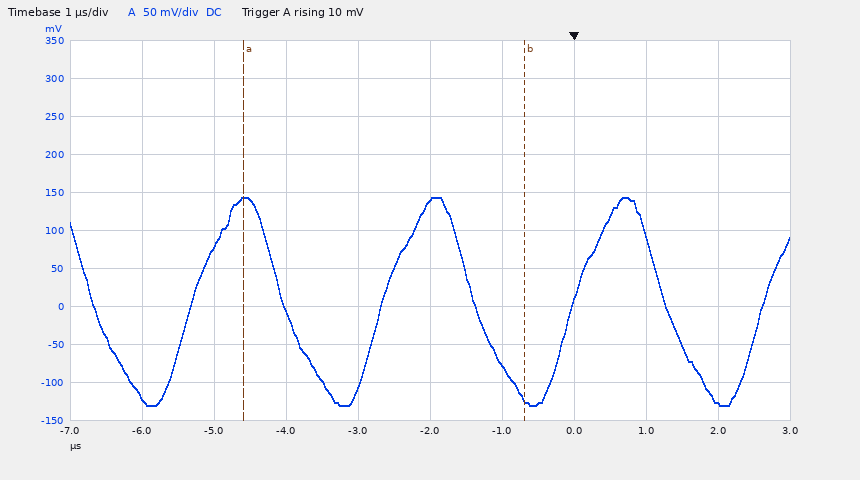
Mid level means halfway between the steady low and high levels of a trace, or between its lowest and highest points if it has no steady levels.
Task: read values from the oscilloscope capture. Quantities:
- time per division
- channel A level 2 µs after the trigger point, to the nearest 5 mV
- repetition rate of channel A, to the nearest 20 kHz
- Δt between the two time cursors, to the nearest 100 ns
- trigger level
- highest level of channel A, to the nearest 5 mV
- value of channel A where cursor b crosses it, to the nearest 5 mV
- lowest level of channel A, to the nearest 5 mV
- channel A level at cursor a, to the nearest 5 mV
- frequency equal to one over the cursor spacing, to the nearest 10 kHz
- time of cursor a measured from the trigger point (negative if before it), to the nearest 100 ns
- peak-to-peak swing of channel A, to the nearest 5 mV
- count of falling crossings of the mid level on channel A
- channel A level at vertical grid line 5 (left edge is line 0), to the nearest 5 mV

1 µs
-130 mV
380 kHz
3.9 µs
10 mV
145 mV
-120 mV
-130 mV
140 mV
260 kHz
-4.6 µs
275 mV
4
140 mV
